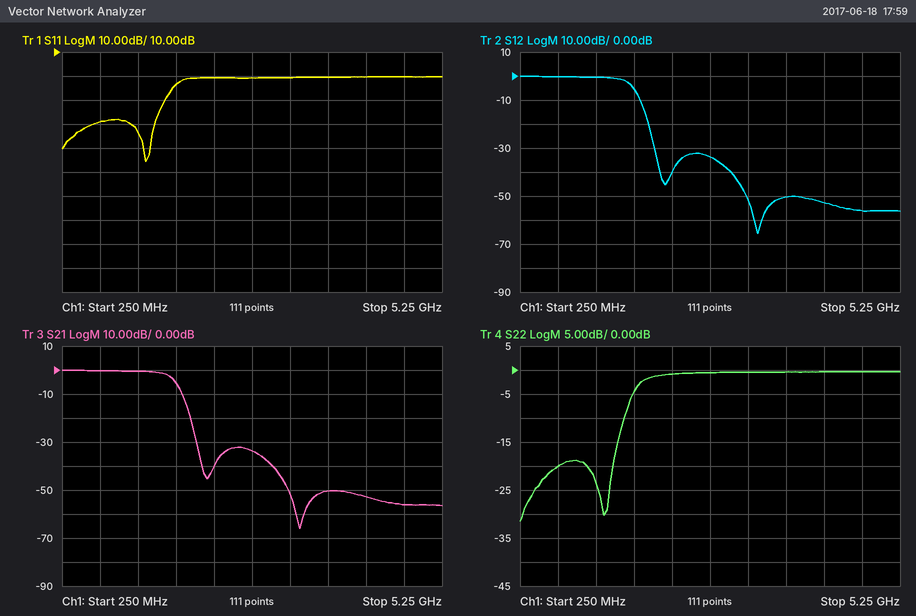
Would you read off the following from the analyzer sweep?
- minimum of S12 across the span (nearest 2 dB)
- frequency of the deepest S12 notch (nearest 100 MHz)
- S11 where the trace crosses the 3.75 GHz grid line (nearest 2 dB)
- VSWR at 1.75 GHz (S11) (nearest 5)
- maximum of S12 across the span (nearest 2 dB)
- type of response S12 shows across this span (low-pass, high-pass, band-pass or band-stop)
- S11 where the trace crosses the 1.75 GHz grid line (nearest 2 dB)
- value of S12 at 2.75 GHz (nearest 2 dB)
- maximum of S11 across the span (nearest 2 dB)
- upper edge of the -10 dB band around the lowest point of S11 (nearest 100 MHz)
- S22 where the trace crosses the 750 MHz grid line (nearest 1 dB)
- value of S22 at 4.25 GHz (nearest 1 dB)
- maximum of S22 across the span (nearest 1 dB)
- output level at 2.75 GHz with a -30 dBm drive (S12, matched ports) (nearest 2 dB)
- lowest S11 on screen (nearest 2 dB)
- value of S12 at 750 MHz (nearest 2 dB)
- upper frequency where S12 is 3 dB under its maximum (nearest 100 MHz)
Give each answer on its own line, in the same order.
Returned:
-66 dB
3.4 GHz
0 dB
5
0 dB
low-pass
-4 dB
-34 dB
0 dB
1.6 GHz
-20 dB
0 dB
0 dB
-64 dBm
-36 dB
0 dB
1.7 GHz
